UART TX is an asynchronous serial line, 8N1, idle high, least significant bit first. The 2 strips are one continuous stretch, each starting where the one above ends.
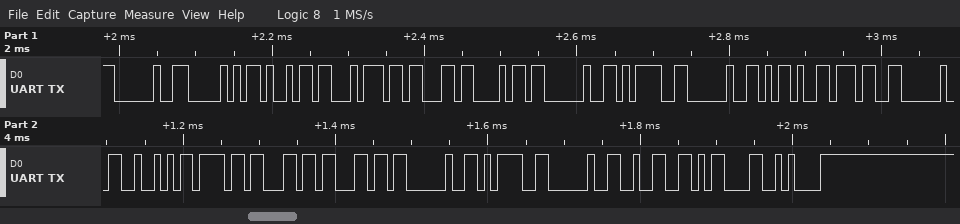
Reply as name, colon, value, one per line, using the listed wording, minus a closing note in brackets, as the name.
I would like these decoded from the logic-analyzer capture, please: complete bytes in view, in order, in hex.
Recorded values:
complete bytes in view, in order, in hex: 0x20 0x50 0x69 0x74 0x63 0x68 0x20 0x3D 0x20 0x2D 0x37 0x20 0x52 0x6F 0x6C 0x6C 0x20 0x3D 0x20 0x32 0x0D 0x0A
